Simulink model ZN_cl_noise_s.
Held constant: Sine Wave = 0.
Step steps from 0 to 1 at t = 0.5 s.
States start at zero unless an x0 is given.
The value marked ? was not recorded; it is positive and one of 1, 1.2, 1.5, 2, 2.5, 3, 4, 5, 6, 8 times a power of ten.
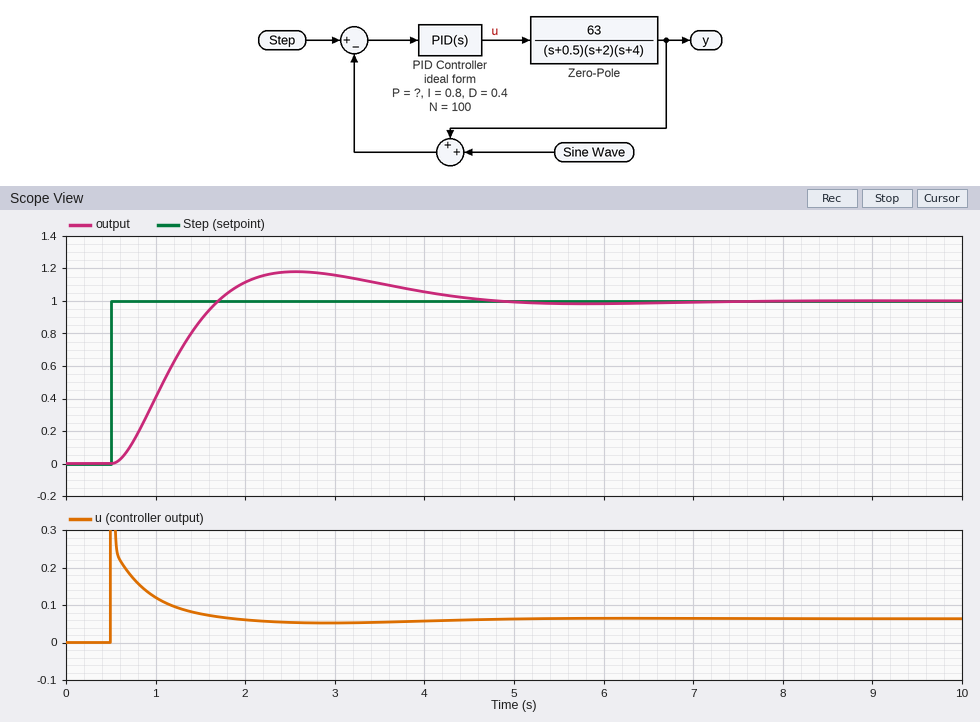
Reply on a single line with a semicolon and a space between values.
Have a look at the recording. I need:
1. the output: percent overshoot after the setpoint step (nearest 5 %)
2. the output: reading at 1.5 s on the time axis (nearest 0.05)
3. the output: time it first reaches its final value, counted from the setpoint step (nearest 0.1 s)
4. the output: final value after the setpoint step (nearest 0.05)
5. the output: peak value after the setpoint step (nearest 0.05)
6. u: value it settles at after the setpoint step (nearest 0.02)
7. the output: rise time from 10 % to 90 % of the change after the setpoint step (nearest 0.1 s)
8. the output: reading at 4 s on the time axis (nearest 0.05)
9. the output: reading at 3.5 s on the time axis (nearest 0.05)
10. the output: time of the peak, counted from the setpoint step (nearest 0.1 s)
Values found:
20 %; 0.90; 1.2 s; 1.00; 1.20; 0.06; 0.8 s; 1.05; 1.10; 2.1 s
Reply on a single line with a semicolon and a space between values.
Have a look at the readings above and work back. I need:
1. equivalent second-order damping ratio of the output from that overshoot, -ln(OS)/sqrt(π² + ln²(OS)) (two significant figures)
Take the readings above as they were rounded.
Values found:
0.46
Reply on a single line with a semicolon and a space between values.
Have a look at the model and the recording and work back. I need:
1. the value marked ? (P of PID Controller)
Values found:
0.25
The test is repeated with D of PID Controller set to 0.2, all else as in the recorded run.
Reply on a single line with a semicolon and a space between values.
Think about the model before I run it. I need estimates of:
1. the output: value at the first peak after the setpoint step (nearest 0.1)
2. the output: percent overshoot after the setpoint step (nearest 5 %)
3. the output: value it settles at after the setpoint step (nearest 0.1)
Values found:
1.3; 35 %; 1.0
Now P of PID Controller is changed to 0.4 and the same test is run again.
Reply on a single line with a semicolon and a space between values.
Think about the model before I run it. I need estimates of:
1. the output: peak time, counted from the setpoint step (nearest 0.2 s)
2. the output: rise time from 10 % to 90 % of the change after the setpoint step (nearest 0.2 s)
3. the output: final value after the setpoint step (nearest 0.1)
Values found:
1.4 s; 0.6 s; 1.0
